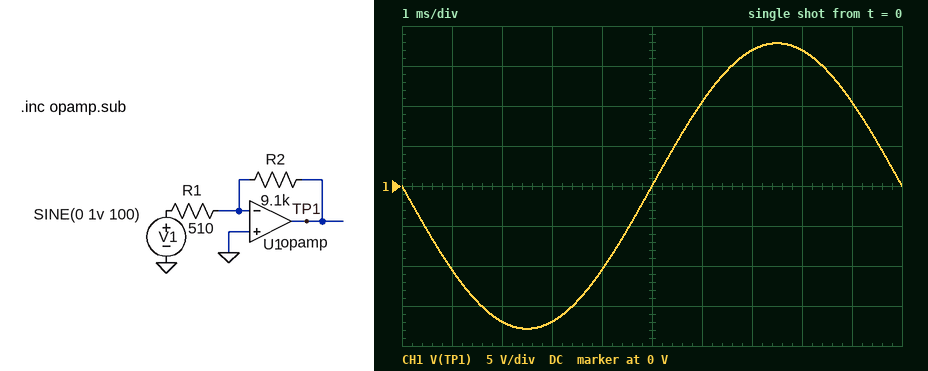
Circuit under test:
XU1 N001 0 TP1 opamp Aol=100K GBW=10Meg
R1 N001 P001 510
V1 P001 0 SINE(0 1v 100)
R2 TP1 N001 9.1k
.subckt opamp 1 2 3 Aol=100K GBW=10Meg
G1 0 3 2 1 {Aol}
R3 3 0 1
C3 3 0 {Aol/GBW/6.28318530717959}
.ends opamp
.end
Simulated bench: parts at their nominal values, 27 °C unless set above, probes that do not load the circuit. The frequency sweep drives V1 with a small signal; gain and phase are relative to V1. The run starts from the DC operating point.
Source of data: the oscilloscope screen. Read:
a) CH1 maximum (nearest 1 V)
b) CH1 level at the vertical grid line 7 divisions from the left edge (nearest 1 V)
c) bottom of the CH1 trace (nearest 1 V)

18 V
17 V
-18 V
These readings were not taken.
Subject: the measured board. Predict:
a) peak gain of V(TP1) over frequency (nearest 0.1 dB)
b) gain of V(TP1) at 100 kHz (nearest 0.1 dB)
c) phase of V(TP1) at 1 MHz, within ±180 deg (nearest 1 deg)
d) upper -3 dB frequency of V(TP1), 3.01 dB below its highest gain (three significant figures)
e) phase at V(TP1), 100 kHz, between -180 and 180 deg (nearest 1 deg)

25.0 dB
24.9 dB
118 deg
531 kHz
169 deg
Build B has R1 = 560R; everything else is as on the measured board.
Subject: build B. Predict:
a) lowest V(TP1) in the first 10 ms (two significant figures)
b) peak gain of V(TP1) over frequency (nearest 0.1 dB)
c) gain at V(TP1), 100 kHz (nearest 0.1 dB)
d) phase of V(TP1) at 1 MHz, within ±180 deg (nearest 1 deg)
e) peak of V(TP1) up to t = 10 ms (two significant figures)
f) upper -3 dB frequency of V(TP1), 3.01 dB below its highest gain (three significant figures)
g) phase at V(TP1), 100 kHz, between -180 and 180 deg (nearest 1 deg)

-16 V
24.2 dB
24.1 dB
120 deg
16 V
580 kHz
170 deg
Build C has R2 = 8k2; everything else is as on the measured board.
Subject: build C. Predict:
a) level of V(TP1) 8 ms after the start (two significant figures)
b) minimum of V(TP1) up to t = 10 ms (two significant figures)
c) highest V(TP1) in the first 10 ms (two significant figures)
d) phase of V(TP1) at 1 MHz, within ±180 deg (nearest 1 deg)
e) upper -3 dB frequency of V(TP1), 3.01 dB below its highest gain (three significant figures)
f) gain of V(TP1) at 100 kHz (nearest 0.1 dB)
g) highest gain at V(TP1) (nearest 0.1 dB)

15 V
-16 V
16 V
120 deg
586 kHz
24.0 dB
24.1 dB
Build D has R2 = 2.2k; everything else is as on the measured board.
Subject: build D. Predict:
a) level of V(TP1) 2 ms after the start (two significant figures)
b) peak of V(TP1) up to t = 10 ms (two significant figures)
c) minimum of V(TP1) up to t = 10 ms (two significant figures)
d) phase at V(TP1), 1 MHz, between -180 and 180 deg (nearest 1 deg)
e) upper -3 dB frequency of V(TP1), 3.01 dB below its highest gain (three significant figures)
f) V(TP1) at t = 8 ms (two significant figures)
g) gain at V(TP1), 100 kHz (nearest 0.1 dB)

-4.1 V
4.3 V
-4.3 V
152 deg
1.88 MHz
4.1 V
12.7 dB
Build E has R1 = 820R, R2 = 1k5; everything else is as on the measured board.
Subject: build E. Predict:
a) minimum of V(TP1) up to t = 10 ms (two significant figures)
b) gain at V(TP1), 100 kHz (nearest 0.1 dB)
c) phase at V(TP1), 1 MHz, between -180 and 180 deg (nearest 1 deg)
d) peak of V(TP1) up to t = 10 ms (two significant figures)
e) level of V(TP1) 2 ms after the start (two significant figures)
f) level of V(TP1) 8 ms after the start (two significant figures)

-1.8 V
5.2 dB
164 deg
1.8 V
-1.7 V
1.7 V
